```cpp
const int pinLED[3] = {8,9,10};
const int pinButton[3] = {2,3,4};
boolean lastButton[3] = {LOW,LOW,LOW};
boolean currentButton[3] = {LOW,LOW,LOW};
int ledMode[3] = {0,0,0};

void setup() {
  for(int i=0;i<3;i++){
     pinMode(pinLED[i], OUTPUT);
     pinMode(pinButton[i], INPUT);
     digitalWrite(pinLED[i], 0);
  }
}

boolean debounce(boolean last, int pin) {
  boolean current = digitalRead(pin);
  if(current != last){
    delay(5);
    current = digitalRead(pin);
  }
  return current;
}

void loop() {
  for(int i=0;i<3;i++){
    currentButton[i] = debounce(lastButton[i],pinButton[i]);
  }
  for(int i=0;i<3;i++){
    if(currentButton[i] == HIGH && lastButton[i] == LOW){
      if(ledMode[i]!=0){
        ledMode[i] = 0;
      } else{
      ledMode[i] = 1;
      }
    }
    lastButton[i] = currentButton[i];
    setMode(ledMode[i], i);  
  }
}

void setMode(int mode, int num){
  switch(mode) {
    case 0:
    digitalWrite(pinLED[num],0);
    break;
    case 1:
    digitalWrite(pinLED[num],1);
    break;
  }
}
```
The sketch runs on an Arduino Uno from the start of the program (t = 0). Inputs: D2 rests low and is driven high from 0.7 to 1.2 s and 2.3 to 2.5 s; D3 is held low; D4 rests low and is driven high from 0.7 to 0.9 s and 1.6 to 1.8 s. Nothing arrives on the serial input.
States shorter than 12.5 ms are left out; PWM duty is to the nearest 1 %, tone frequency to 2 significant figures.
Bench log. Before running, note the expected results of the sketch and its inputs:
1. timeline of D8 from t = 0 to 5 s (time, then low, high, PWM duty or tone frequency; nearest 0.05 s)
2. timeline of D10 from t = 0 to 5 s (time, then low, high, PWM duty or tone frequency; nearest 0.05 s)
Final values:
0 s low; 0.7 s high; 2.3 s low
0 s low; 0.7 s high; 1.6 s low
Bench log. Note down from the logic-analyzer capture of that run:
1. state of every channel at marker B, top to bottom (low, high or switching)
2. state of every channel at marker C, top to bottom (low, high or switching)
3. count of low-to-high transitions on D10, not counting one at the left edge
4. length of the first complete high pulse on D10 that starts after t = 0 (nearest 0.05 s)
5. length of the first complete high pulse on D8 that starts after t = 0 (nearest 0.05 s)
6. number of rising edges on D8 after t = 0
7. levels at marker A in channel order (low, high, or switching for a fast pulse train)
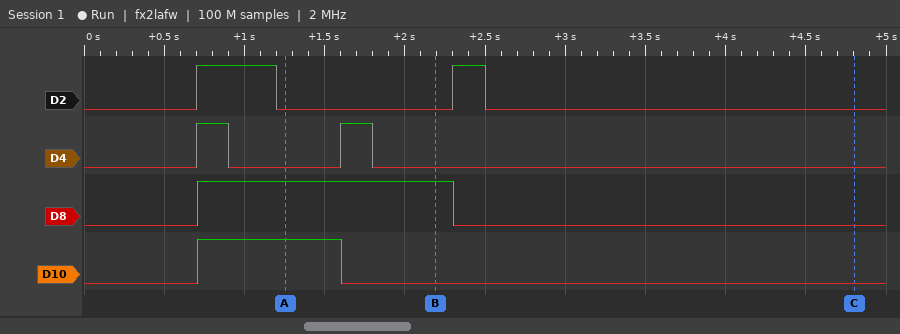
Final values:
D2 low, D4 low, D8 high, D10 low
D2 low, D4 low, D8 low, D10 low
1
0.90 s
1.60 s
1
D2 low, D4 low, D8 high, D10 high
